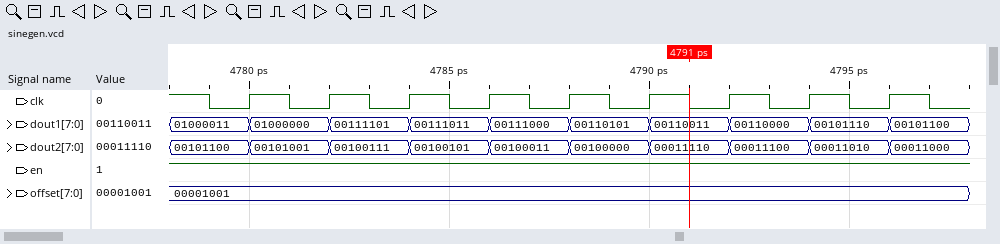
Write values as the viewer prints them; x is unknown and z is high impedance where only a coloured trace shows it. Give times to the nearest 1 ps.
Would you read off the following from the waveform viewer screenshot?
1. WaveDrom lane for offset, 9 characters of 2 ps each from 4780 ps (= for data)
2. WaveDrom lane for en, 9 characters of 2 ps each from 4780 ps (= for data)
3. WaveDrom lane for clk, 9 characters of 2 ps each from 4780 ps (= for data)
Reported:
{name: 'offset', wave: '=........', data: '00001001'}
{name: 'en', wave: '1........'}
{name: 'clk', wave: 'p........'}
